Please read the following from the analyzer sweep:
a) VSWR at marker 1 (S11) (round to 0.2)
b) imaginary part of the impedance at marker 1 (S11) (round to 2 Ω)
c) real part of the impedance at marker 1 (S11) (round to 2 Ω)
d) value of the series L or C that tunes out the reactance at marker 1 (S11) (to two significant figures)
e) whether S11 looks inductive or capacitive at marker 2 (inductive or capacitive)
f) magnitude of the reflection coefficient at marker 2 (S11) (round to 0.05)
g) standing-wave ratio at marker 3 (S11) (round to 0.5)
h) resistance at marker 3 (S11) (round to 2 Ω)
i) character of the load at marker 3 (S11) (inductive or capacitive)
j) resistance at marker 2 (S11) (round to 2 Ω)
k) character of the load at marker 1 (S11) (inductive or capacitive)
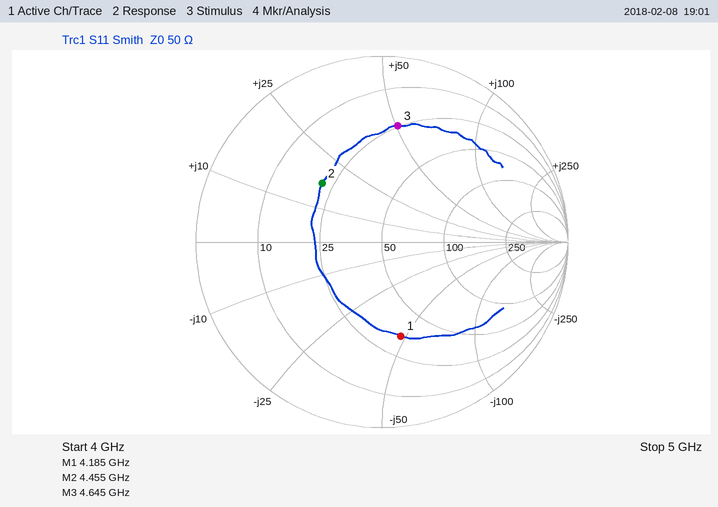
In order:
3.2
-48 Ω
34 Ω
1.8 nH
inductive
0.45
4.5
24 Ω
inductive
22 Ω
capacitive
